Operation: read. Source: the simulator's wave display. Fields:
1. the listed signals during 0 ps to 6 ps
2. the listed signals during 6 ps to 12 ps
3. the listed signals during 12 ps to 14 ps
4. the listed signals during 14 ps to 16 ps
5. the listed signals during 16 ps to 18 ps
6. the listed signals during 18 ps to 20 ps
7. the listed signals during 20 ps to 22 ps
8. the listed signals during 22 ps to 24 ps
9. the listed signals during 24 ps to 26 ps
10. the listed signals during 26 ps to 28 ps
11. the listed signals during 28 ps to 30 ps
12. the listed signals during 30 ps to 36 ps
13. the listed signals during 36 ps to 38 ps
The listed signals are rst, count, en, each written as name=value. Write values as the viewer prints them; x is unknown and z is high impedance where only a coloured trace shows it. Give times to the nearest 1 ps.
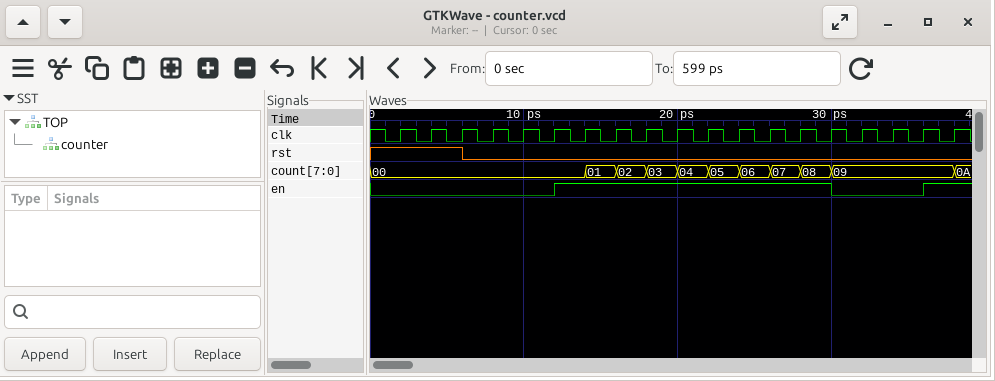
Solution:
rst=1, count=00, en=0
rst=0, count=00, en=0
rst=0, count=00, en=1
rst=0, count=01, en=1
rst=0, count=02, en=1
rst=0, count=03, en=1
rst=0, count=04, en=1
rst=0, count=05, en=1
rst=0, count=06, en=1
rst=0, count=07, en=1
rst=0, count=08, en=1
rst=0, count=09, en=0
rst=0, count=09, en=1
